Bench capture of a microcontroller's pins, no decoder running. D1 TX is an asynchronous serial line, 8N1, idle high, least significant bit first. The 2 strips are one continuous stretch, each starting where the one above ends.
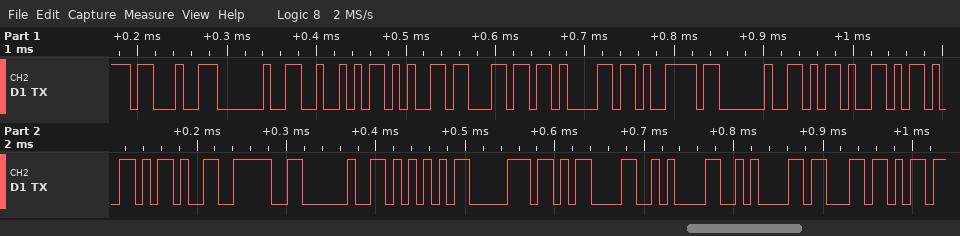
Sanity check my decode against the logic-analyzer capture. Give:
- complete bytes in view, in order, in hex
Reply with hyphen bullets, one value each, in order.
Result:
- 23 20 52 65 6C 61 79 20 2D 2D 2D 3E 20 55 70 0D 0A 0A 63
